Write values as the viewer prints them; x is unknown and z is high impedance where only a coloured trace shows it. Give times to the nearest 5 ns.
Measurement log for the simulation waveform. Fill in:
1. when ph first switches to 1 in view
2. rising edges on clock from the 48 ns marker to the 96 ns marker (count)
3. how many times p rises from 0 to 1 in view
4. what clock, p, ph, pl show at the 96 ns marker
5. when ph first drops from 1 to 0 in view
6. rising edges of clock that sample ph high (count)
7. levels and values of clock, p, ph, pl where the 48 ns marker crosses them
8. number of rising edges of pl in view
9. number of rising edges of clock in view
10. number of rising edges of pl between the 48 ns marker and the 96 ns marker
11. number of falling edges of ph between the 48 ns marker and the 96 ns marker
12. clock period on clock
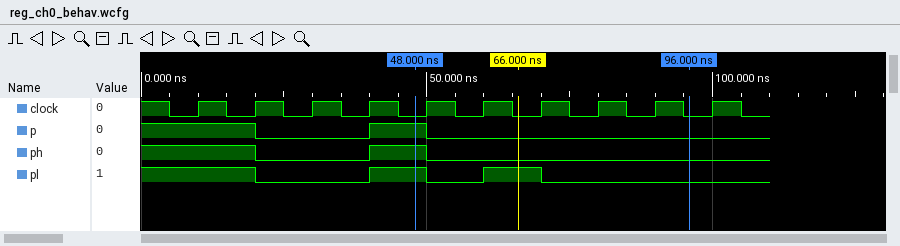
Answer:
40 ns
5
1
clock=0, p=0, ph=0, pl=0
20 ns
3
clock=0, p=1, ph=1, pl=1
2
10
1
1
10 ns
